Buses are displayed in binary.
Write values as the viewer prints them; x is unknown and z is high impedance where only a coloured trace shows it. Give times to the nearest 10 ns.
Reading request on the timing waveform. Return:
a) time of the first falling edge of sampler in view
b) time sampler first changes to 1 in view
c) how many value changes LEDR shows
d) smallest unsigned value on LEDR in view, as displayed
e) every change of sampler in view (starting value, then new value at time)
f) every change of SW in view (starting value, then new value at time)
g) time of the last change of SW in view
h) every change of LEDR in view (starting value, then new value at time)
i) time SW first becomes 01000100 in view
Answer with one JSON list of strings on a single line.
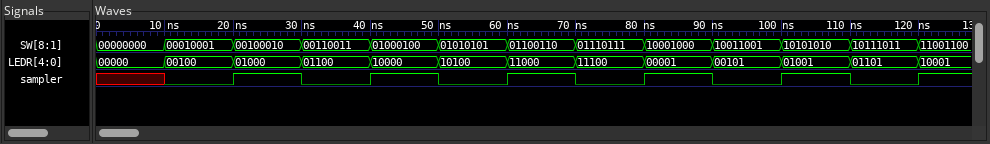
["30 ns", "20 ns", "12", "00000", "x, 0 at 10 ns, 1 at 20 ns, 0 at 30 ns, 1 at 40 ns, 0 at 50 ns, 1 at 60 ns, 0 at 70 ns, 1 at 80 ns, 0 at 90 ns, 1 at 100 ns, 0 at 110 ns, 1 at 120 ns", "00000000, 00010001 at 10 ns, 00100010 at 20 ns, 00110011 at 30 ns, 01000100 at 40 ns, 01010101 at 50 ns, 01100110 at 60 ns, 01110111 at 70 ns, 10001000 at 80 ns, 10011001 at 90 ns, 10101010 at 100 ns, 10111011 at 110 ns, 11001100 at 120 ns", "120 ns", "00000, 00100 at 10 ns, 01000 at 20 ns, 01100 at 30 ns, 10000 at 40 ns, 10100 at 50 ns, 11000 at 60 ns, 11100 at 70 ns, 00001 at 80 ns, 00101 at 90 ns, 01001 at 100 ns, 01101 at 110 ns, 10001 at 120 ns", "40 ns"]
